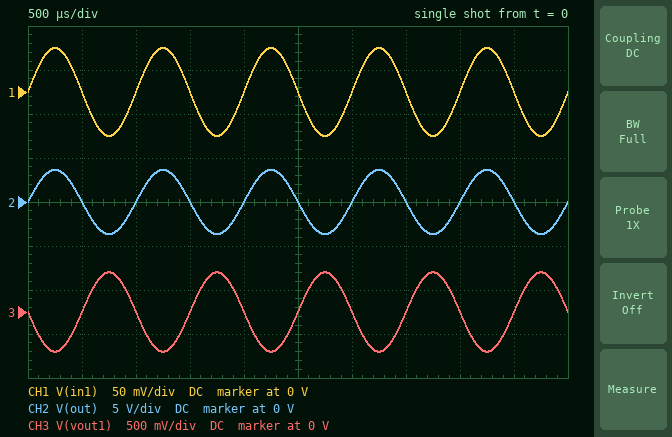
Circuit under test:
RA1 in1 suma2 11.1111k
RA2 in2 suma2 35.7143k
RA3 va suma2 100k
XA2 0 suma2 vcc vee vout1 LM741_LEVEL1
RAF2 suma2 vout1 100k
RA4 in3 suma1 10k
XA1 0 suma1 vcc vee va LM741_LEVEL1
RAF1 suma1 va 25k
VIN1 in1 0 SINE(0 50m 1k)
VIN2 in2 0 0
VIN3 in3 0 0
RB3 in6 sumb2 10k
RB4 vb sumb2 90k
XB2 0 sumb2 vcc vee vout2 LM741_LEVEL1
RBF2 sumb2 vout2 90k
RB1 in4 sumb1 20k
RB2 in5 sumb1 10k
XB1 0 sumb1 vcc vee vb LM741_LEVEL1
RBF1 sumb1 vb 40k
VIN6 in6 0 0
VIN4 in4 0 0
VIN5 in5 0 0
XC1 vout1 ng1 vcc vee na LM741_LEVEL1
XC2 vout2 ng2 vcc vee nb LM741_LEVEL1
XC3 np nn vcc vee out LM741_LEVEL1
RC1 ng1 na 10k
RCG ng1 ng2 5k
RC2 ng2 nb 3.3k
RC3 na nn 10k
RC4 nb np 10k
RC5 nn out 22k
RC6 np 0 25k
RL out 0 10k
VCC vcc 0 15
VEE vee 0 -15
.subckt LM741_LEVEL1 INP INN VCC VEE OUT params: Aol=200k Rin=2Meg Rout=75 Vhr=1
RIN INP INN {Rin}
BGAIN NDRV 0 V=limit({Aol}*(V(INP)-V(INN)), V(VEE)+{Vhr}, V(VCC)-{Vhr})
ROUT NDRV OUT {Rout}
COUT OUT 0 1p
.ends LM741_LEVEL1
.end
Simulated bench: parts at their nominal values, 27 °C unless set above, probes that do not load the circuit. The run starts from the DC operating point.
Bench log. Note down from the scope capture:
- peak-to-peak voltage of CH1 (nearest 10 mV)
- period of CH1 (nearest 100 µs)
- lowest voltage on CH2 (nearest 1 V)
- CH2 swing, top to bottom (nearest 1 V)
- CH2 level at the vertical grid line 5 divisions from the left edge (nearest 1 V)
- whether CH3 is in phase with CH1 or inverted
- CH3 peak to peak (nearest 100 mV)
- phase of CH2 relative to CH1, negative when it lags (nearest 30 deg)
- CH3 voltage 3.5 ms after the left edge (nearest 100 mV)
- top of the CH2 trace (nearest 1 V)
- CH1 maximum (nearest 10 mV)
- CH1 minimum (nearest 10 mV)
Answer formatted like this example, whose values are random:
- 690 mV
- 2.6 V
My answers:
- 100 mV
- 1.0 ms
- -4 V
- 7 V
- 0 V
- inverted
- 900 mV
- 0 deg
- 0 V
- 4 V
- 50 mV
- -50 mV
